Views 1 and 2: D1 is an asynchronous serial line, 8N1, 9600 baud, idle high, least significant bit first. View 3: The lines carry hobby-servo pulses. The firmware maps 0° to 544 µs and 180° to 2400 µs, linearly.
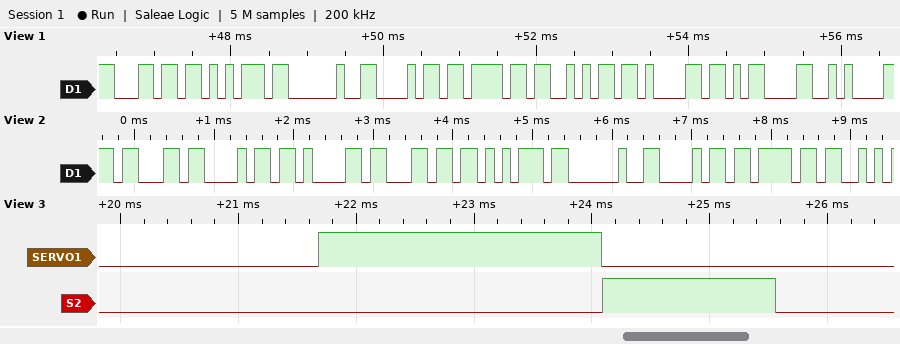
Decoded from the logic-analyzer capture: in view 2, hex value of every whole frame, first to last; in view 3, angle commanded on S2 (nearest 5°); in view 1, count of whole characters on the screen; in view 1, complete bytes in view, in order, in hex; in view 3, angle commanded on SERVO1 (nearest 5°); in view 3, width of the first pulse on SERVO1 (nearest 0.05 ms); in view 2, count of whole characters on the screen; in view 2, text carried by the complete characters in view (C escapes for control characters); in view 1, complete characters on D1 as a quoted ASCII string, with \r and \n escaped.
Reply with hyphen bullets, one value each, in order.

- 63 68 61 6C 75 20 68 6F
- 90°
- 9
- 6C 75 20 68 6F 6A 61 0D 0A
- 180°
- 2.40 ms
- 8
- "chalu ho"
- "lu hoja\r\n"
